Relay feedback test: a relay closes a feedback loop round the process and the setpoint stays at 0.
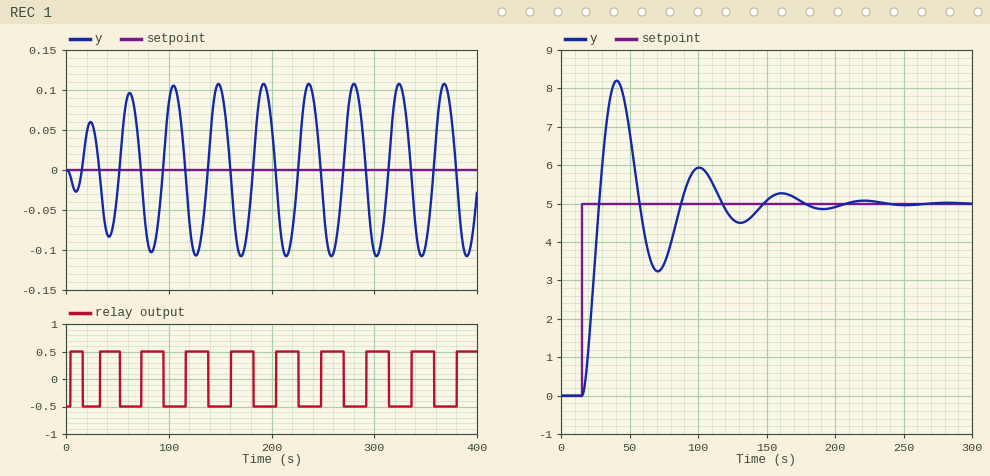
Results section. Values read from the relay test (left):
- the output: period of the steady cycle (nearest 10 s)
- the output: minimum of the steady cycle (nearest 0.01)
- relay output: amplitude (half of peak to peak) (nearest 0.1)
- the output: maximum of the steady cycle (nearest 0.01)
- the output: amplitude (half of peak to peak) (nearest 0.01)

40 s
-0.11
0.5
0.11
0.11
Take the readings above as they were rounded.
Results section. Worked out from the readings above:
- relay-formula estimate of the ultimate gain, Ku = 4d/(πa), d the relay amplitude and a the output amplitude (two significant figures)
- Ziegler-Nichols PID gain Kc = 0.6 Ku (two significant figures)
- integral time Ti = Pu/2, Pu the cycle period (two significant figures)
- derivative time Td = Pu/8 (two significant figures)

5.8
3.5
20 s
5.0 s
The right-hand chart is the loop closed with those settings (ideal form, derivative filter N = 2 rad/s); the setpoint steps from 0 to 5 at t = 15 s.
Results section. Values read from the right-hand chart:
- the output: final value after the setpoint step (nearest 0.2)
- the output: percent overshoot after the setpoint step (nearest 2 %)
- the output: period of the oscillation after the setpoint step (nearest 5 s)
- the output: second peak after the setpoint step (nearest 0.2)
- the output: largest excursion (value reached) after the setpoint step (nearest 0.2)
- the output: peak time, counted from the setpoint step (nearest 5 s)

5.0
64 %
60 s
6.0
8.2
25 s
